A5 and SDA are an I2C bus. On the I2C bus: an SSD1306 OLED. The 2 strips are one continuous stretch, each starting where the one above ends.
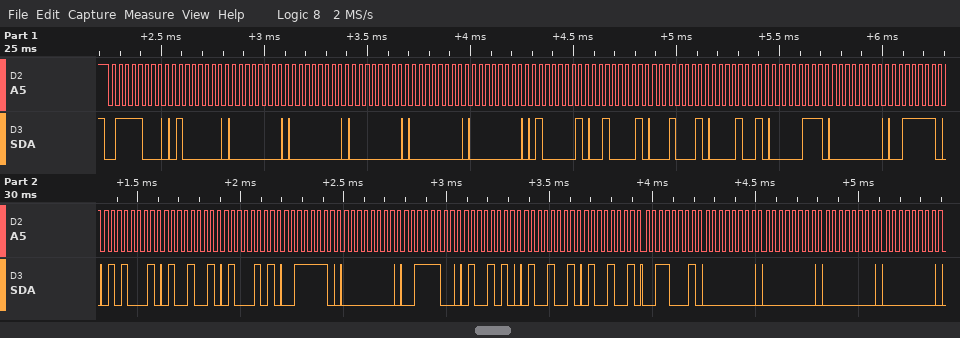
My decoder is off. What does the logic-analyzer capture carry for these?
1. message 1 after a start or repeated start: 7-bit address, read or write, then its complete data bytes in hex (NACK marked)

0x3C write: 40 00 00 00 00 00 41 21 11 09 07 00 3E 51 49 45 3E 00 3C 4A 49 49 31 00 00 00 00
